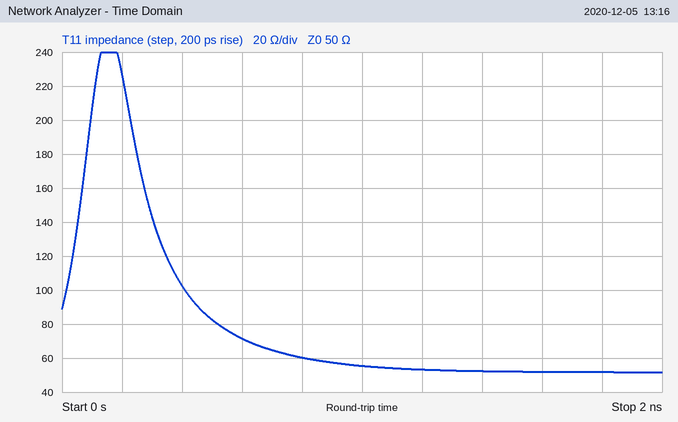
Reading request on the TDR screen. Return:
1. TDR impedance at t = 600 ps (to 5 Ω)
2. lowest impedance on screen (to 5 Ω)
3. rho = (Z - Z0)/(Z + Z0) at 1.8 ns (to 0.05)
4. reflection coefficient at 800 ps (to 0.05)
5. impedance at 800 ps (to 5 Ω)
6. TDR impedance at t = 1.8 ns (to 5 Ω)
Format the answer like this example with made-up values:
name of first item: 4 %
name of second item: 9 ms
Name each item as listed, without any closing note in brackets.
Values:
TDR impedance at t = 600 ps: 70 Ω
lowest impedance on screen: 50 Ω
rho = (Z - Z0)/(Z + Z0) at 1.8 ns: 0.00
reflection coefficient at 800 ps: +0.10
impedance at 800 ps: 60 Ω
TDR impedance at t = 1.8 ns: 50 Ω
